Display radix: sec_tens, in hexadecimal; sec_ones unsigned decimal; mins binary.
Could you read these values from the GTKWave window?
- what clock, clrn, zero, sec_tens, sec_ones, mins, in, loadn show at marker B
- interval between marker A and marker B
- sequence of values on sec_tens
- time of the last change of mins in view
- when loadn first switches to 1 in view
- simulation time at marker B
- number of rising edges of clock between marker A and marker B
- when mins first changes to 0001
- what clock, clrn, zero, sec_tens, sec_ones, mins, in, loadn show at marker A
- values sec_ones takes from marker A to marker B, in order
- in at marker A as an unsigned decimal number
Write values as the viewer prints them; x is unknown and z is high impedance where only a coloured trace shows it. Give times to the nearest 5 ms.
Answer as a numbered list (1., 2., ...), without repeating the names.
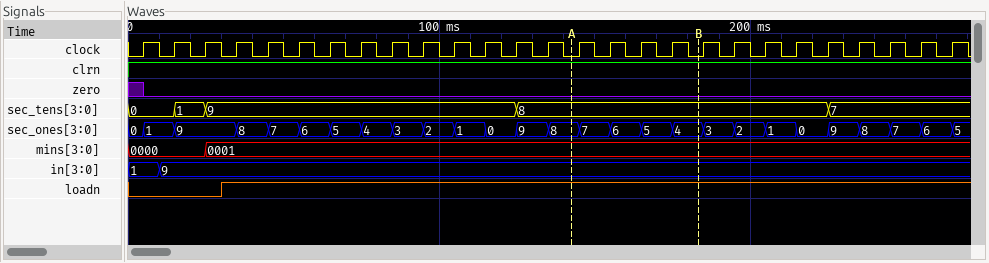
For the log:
1. clock=0, clrn=1, zero=0, sec_tens=8, sec_ones=4, mins=0001, in=9, loadn=1
2. 40 ms
3. 0, 1, 9, 8, 7
4. 25 ms
5. 30 ms
6. 185 ms
7. 4
8. 25 ms
9. clock=0, clrn=1, zero=0, sec_tens=8, sec_ones=8, mins=0001, in=9, loadn=1
10. 8, 7, 6, 5, 4
11. 9
